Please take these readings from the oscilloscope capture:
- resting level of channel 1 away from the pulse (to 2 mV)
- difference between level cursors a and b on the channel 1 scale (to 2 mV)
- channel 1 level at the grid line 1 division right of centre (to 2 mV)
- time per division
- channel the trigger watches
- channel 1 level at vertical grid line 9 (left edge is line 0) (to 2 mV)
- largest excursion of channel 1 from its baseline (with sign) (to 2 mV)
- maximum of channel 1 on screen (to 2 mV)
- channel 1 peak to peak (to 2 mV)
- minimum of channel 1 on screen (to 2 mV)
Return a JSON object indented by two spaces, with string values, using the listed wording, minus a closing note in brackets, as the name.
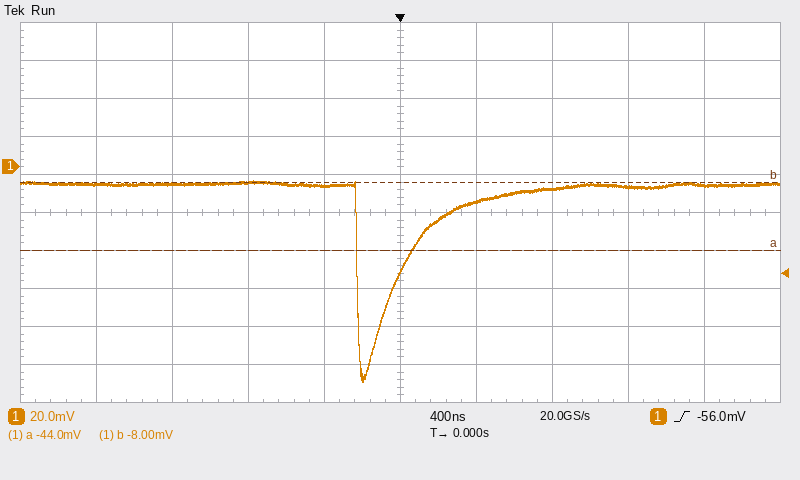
{
  "resting level of channel 1 away from the pulse": "-10 mV",
  "difference between level cursors a and b on the channel 1 scale": "36 mV",
  "channel 1 level at the grid line 1 division right of centre": "-18 mV",
  "time per division": "400 ns",
  "channel the trigger watches": "channel 1",
  "channel 1 level at vertical grid line 9 (left edge is line 0)": "-10 mV",
  "largest excursion of channel 1 from its baseline (with sign)": "-104 mV",
  "maximum of channel 1 on screen": "-8 mV",
  "channel 1 peak to peak": "106 mV",
  "minimum of channel 1 on screen": "-114 mV"
}
